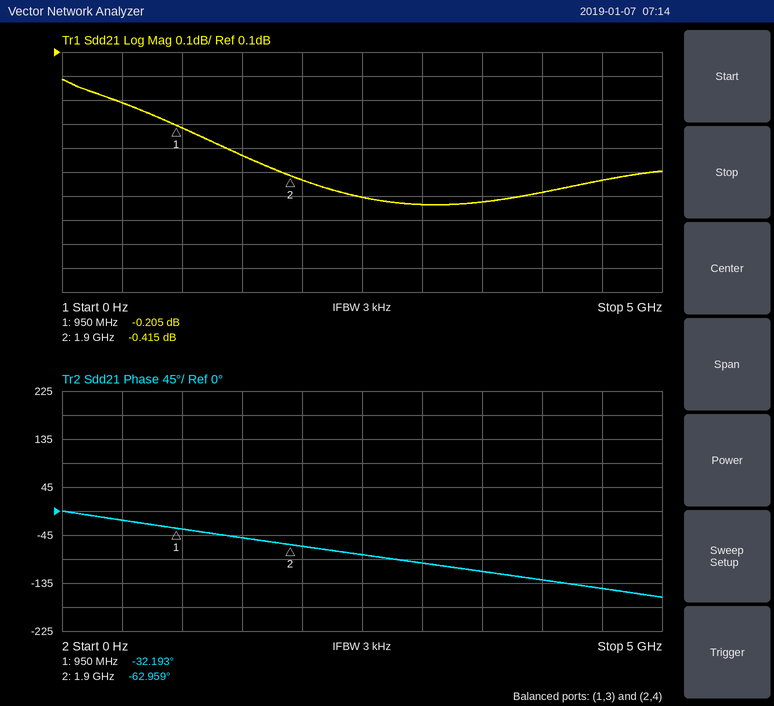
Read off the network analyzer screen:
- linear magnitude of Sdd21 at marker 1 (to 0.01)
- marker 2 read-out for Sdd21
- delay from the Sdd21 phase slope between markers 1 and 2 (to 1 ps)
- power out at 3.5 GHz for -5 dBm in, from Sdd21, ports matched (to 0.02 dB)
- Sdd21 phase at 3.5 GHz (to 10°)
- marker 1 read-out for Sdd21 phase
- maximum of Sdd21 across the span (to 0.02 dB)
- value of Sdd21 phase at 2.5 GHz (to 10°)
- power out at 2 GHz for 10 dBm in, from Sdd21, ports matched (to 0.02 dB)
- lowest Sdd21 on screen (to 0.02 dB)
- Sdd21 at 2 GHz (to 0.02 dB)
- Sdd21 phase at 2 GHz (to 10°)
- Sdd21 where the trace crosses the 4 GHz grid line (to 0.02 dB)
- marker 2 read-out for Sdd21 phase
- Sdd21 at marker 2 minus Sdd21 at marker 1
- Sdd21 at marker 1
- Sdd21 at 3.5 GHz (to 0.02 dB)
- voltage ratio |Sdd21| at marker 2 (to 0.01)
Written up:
0.98
-0.415 dB
90 ps
-5.52 dBm
-110°
-32.193°
-0.02 dB
-80°
9.56 dBm
-0.54 dB
-0.44 dB
-70°
-0.48 dB
-62.959°
-0.210 dB
-0.205 dB
-0.52 dB
0.95
